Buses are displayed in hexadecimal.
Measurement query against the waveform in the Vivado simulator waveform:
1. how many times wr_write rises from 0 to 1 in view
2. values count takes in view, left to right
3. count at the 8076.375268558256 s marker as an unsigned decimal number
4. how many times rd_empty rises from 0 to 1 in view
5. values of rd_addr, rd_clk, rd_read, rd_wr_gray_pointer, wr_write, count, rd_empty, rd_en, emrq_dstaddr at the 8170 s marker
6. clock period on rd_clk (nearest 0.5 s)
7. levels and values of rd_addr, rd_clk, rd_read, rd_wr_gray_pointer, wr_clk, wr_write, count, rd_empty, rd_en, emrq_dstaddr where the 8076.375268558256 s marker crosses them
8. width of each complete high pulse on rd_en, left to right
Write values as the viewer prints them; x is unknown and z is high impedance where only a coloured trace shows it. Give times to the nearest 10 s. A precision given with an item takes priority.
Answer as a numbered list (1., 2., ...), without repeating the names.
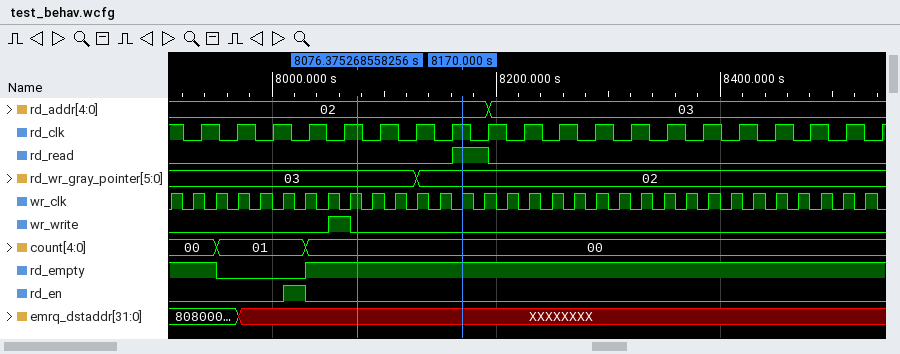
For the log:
1. 1
2. 00, 01, 00
3. 0
4. 1
5. rd_addr=02, rd_clk=1, rd_read=1, rd_wr_gray_pointer=02, wr_write=0, count=00, rd_empty=1, rd_en=0, emrq_dstaddr=XXXXXXXX
6. 32 s
7. rd_addr=02, rd_clk=1, rd_read=0, rd_wr_gray_pointer=03, wr_clk=1, wr_write=0, count=00, rd_empty=1, rd_en=0, emrq_dstaddr=XXXXXXXX
8. 20 s
